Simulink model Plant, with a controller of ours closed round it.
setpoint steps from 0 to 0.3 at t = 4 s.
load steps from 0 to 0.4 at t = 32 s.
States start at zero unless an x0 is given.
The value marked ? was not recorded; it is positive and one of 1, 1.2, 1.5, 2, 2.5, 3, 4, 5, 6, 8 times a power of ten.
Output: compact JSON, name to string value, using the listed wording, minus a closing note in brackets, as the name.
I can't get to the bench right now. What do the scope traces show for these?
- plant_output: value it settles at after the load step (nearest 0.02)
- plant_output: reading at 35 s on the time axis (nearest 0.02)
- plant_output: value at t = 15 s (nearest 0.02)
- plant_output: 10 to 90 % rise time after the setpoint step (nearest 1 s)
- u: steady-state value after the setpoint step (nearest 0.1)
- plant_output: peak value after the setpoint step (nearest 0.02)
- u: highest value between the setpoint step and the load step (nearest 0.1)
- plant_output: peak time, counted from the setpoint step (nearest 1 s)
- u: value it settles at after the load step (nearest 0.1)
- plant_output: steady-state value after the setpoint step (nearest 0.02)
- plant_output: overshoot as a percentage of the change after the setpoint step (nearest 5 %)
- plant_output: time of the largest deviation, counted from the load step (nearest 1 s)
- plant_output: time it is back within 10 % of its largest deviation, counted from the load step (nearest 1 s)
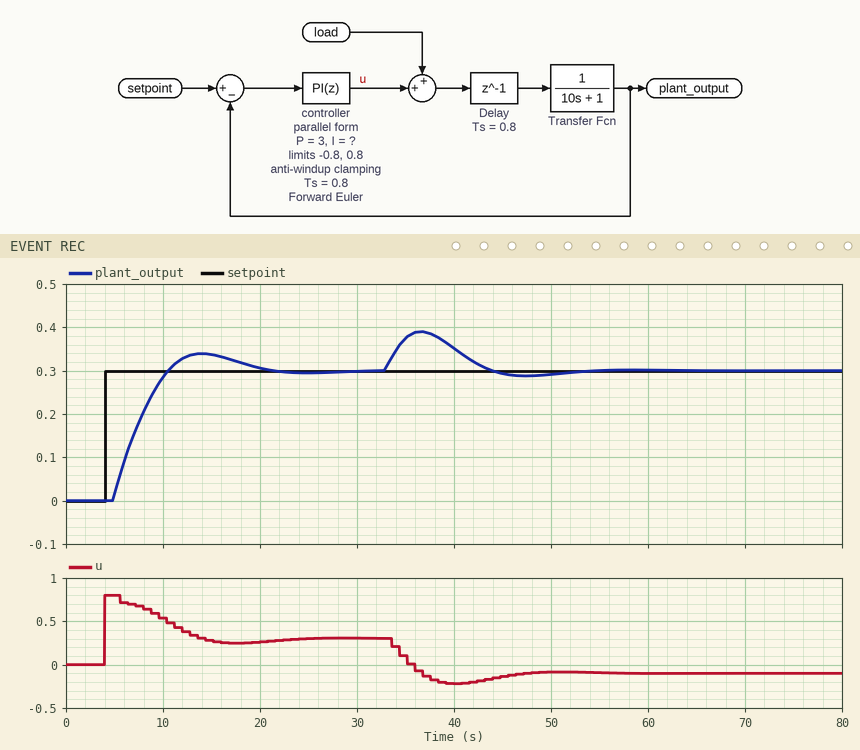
{"plant_output: value it settles at after the load step": "0.30", "plant_output: reading at 35 s on the time axis": "0.38", "plant_output: value at t = 15 s": "0.34", "plant_output: 10 to 90 % rise time after the setpoint step": "4 s", "u: steady-state value after the setpoint step": "0.3", "plant_output: peak value after the setpoint step": "0.34", "u: highest value between the setpoint step and the load step": "0.8", "plant_output: peak time, counted from the setpoint step": "10 s", "u: value it settles at after the load step": "-0.1", "plant_output: steady-state value after the setpoint step": "0.30", "plant_output: overshoot as a percentage of the change after the setpoint step": "15 %", "plant_output: time of the largest deviation, counted from the load step": "5 s", "plant_output: time it is back within 10 % of its largest deviation, counted from the load step": "18 s"}
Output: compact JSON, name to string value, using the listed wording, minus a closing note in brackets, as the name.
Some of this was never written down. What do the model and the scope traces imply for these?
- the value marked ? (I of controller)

{"the value marked ?": "0.8"}
